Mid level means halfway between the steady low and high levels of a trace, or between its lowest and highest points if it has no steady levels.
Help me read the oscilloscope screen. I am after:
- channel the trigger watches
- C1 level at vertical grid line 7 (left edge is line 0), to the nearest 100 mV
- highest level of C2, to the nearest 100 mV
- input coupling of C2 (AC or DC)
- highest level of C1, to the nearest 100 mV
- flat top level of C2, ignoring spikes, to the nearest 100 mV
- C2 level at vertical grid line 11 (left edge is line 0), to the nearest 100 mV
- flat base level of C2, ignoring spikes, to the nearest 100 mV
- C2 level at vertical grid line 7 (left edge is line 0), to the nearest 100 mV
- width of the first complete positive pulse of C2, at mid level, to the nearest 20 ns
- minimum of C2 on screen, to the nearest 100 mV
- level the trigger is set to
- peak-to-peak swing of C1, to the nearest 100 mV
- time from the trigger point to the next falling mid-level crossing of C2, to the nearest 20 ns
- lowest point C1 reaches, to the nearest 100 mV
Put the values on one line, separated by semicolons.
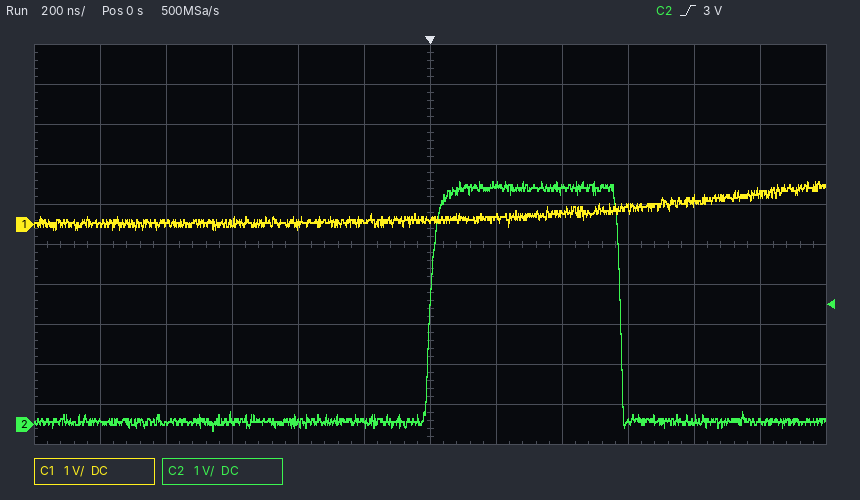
C2; 200 mV; 6.1 V; DC; 1.1 V; 5.9 V; 100 mV; 100 mV; 6.0 V; 580 ns; -200 mV; 3 V; 1.2 V; 580 ns; -100 mV
